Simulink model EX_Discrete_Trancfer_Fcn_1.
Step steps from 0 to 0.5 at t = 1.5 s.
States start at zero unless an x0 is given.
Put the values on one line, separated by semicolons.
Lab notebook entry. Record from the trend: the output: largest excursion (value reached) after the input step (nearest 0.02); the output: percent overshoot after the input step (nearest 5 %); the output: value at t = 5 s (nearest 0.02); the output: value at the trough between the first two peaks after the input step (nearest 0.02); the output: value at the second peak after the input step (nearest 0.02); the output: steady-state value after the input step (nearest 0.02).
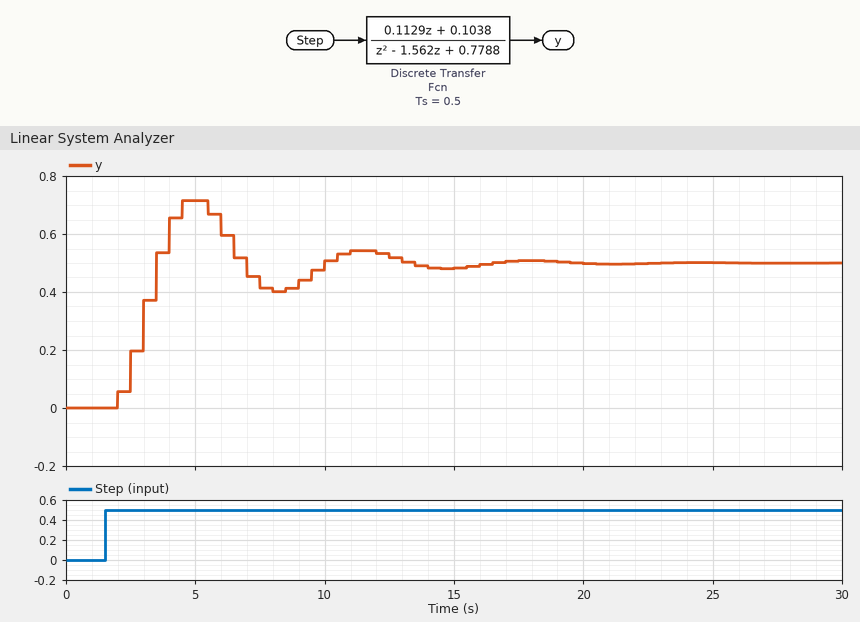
0.72; 45 %; 0.72; 0.40; 0.54; 0.50
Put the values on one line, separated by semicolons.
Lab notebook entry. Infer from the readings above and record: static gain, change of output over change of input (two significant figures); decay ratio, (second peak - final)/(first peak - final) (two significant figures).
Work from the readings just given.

1.0; 0.18
